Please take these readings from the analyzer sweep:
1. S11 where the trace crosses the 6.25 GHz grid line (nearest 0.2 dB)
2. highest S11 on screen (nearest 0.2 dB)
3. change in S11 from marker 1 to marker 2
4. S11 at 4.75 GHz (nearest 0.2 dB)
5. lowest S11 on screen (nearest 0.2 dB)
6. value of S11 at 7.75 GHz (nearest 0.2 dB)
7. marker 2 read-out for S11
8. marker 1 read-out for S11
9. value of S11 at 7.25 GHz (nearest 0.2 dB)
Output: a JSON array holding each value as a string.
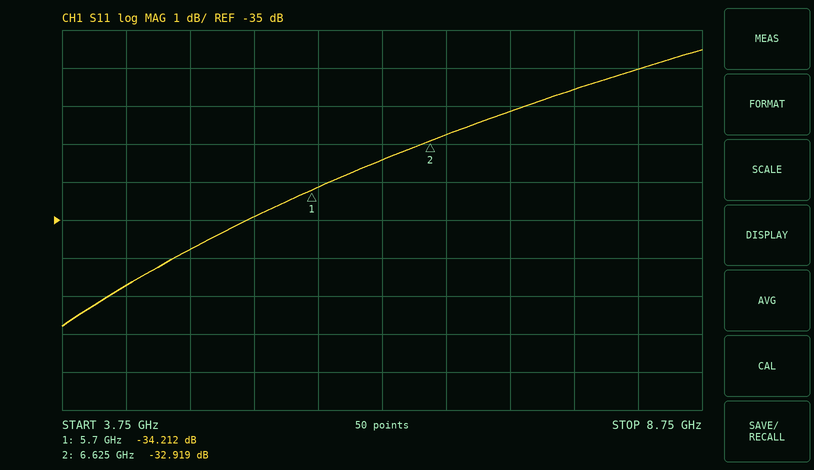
["-33.4 dB", "-30.6 dB", "1.293 dB", "-35.8 dB", "-37.8 dB", "-31.6 dB", "-32.919 dB", "-34.212 dB", "-32.2 dB"]
